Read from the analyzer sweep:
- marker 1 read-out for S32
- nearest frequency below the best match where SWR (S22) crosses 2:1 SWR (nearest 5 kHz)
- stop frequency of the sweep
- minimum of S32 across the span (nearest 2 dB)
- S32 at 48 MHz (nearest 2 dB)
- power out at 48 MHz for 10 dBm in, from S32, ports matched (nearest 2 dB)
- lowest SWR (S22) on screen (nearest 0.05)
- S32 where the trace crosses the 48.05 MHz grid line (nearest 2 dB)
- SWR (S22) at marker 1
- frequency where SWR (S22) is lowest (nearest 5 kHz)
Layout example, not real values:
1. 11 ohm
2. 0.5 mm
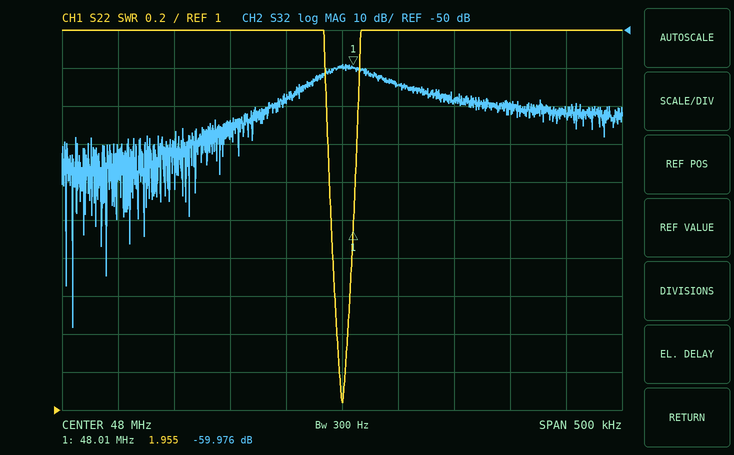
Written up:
1. -59.976 dB
2. 47.990 MHz
3. 48.25 MHz
4. -128 dB
5. -60 dB
6. -50 dBm
7. 1.05
8. -64 dB
9. 1.955
10. 48.000 MHz
